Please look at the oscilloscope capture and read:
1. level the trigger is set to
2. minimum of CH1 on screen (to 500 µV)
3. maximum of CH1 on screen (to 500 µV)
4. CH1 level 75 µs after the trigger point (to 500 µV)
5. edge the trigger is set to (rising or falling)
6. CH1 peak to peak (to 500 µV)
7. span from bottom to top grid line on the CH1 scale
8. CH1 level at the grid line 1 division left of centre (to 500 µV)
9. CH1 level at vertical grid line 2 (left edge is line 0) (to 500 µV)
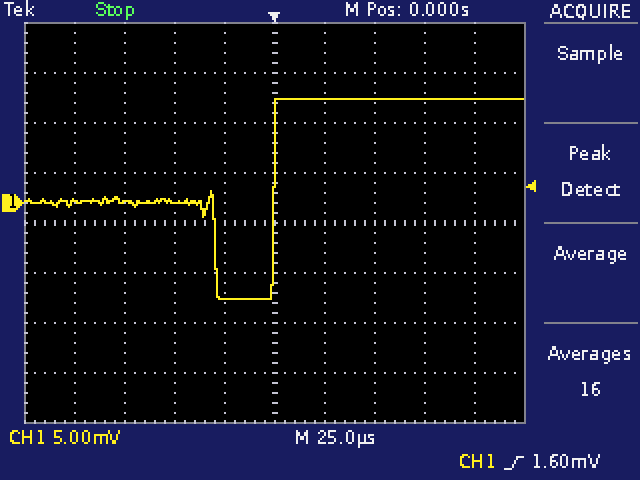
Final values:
1.60 mV
-9.5 mV
10.5 mV
10.5 mV
rising
20.0 mV
40 mV
-9.5 mV
0.0 mV
